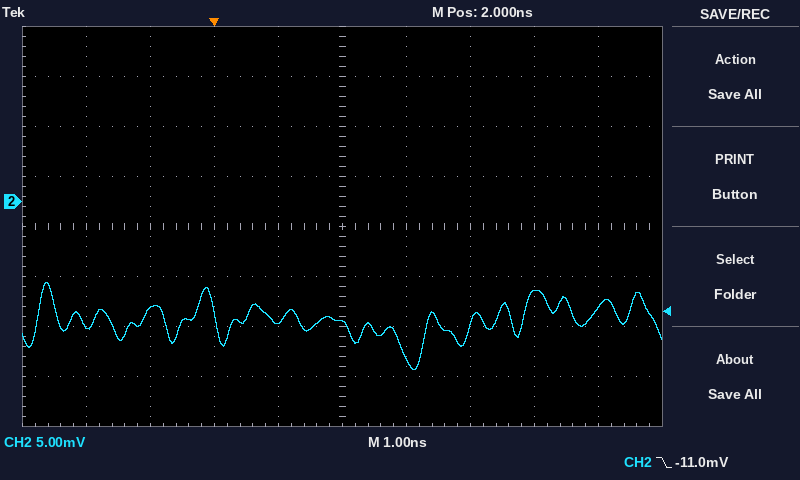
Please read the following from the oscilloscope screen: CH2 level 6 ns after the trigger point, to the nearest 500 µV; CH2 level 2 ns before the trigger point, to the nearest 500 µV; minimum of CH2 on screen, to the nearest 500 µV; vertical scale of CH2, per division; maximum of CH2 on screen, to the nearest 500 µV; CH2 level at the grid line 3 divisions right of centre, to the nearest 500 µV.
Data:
-10.5 mV
-12.5 mV
-17.0 mV
5 mV
-8.0 mV
-9.0 mV
